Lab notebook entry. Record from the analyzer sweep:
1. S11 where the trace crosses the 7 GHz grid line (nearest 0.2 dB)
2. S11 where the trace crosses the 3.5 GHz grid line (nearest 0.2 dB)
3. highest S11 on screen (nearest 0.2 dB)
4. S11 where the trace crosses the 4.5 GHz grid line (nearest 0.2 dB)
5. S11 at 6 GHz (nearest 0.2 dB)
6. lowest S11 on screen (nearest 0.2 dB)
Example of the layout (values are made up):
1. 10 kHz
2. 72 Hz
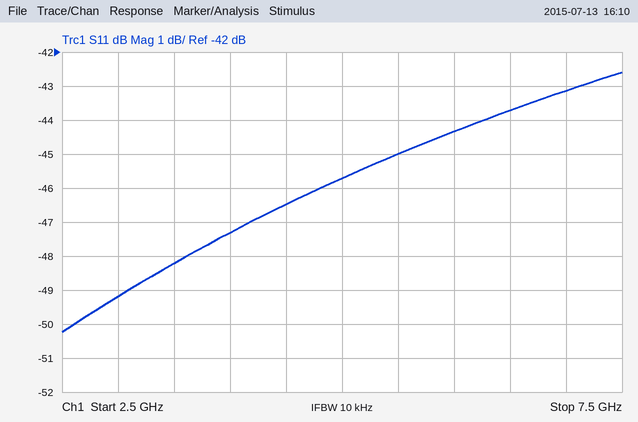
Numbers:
1. -43.2 dB
2. -48.2 dB
3. -42.6 dB
4. -46.4 dB
5. -44.4 dB
6. -50.2 dB
